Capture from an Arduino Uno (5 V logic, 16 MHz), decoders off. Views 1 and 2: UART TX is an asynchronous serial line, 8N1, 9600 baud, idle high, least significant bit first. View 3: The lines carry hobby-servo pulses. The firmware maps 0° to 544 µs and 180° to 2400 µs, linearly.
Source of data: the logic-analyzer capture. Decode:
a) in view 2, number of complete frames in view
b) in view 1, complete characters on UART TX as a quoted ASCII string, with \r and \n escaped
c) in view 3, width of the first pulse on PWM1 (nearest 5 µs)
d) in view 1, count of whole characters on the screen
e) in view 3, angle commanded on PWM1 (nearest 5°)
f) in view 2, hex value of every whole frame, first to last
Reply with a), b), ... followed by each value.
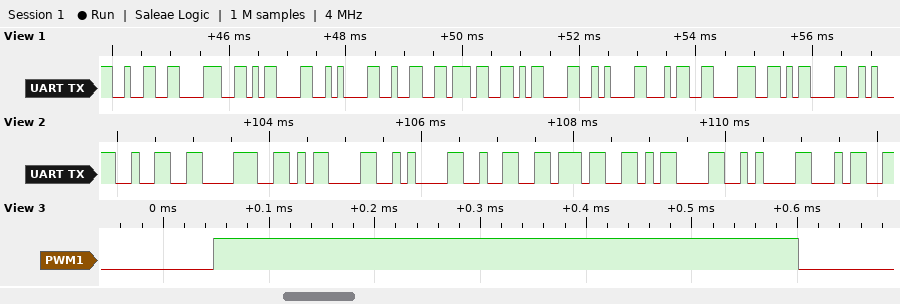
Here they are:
a) 9
b) "28\r\n27\r\n48\r"
c) 555 µs
d) 11
e) 0°
f) 32 38 0D 0A 32 37 0D 0A 34
